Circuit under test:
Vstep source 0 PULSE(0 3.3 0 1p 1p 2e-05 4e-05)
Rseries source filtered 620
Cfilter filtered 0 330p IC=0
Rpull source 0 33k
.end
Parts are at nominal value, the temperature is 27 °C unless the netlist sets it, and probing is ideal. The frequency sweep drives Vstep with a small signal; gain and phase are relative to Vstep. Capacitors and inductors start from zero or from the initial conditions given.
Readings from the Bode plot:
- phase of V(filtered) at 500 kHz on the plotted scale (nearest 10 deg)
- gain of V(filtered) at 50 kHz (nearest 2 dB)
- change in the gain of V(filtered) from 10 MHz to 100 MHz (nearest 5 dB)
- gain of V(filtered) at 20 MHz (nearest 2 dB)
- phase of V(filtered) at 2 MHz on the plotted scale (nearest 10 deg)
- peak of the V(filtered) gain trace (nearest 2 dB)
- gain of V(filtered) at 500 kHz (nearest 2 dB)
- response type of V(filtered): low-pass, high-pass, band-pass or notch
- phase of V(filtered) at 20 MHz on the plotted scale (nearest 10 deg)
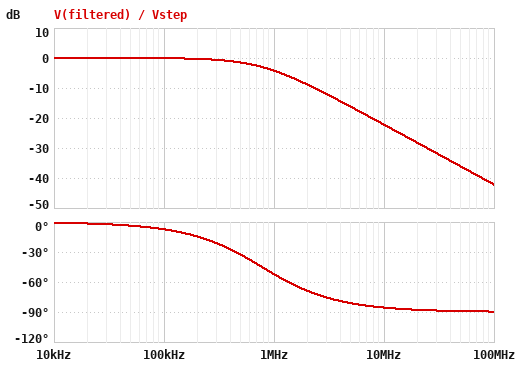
-30 deg
0 dB
-20 dB
-28 dB
-70 deg
0 dB
-2 dB
low-pass
-90 deg
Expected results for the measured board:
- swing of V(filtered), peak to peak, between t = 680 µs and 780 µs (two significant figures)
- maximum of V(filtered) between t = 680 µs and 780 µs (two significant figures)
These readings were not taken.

3.3 V
3.3 V
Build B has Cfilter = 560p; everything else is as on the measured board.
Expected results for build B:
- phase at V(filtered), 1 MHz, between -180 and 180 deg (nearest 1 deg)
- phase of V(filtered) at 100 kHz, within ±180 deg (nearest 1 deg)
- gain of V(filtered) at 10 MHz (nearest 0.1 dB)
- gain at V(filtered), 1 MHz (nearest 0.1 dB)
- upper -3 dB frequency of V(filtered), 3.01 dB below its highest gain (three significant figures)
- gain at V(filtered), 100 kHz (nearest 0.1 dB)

-65 deg
-12 deg
-26.8 dB
-7.6 dB
458 kHz
-0.2 dB
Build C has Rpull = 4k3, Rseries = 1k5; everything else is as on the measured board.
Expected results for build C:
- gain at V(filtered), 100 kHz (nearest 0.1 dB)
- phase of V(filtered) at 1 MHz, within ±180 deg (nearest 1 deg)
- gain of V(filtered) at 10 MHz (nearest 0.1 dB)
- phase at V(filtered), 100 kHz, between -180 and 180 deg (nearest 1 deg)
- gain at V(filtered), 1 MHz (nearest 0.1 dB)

-0.4 dB
-72 deg
-29.9 dB
-17 deg
-10.3 dB
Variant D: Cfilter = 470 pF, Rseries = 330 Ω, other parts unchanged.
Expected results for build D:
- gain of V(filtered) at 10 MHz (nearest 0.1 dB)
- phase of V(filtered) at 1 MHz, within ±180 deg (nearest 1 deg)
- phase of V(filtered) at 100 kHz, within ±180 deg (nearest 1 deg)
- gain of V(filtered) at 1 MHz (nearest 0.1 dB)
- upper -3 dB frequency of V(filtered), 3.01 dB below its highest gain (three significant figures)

-19.8 dB
-44 deg
-6 deg
-2.9 dB
1.03 MHz
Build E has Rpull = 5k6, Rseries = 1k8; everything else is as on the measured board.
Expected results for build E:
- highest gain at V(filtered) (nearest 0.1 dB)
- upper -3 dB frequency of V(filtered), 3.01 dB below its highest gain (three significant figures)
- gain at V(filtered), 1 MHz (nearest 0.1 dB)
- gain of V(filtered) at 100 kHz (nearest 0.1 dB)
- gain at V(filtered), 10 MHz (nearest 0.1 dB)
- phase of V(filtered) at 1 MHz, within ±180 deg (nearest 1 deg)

0 dB
268 kHz
-11.7 dB
-0.6 dB
-31.4 dB
-75 deg
